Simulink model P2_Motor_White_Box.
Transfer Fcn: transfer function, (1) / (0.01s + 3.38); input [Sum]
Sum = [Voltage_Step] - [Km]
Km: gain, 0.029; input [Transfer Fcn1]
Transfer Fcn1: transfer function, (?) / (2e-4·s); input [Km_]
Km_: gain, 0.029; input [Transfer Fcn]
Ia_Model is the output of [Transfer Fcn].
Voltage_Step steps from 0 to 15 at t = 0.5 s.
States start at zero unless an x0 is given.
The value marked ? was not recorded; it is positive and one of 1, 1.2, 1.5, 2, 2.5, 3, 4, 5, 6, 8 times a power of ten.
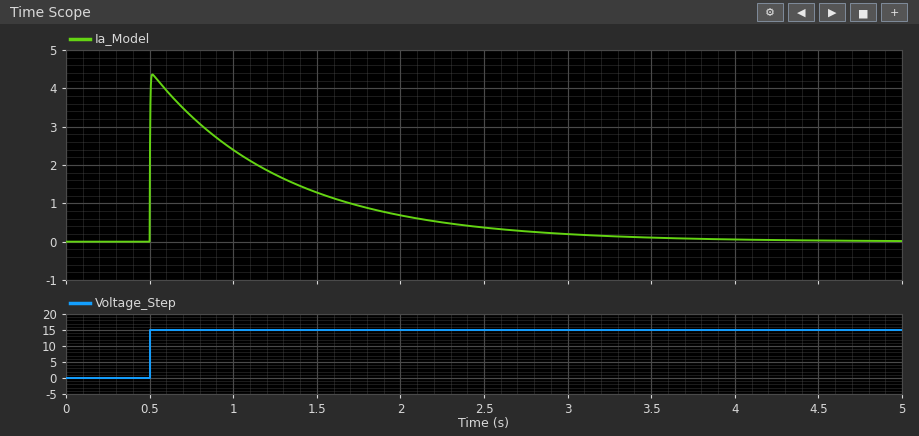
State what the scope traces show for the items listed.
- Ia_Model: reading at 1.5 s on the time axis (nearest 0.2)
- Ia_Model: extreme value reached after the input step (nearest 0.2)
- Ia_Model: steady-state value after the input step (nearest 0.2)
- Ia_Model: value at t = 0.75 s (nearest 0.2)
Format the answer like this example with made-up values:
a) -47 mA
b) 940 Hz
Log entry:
a) 1.2
b) 4.4
c) 0.0
d) 3.2
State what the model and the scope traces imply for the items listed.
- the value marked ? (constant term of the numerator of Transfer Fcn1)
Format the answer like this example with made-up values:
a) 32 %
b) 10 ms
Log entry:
a) 1
